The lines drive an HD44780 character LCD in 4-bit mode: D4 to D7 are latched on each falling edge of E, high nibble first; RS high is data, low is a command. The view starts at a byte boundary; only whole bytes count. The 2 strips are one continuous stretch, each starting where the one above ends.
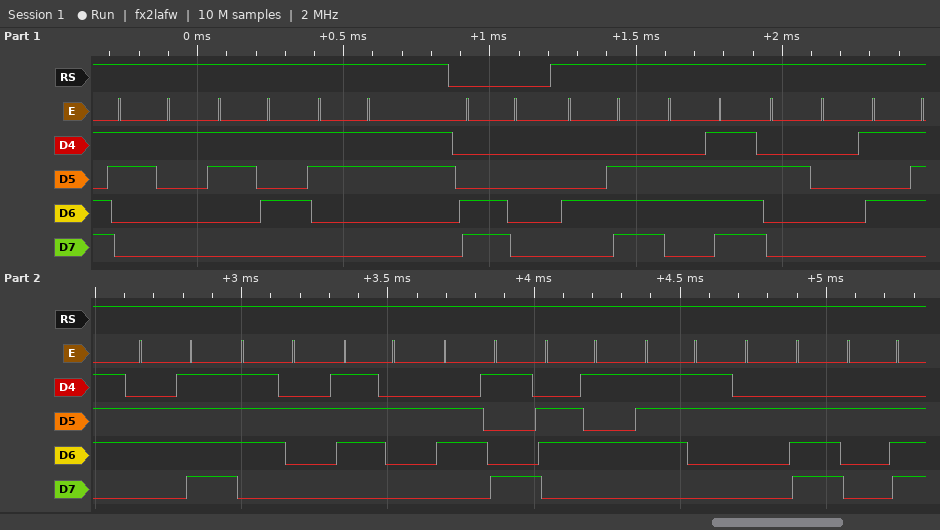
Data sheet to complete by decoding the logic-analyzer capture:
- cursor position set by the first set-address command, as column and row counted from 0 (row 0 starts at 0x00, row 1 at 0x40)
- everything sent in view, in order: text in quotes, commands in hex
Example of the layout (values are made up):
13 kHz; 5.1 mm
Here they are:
column 0, row 1; "153" 0xC0 "No Worries.."
